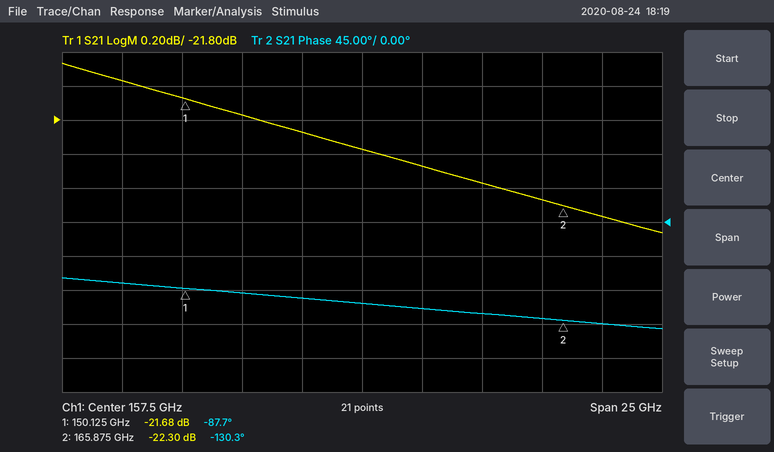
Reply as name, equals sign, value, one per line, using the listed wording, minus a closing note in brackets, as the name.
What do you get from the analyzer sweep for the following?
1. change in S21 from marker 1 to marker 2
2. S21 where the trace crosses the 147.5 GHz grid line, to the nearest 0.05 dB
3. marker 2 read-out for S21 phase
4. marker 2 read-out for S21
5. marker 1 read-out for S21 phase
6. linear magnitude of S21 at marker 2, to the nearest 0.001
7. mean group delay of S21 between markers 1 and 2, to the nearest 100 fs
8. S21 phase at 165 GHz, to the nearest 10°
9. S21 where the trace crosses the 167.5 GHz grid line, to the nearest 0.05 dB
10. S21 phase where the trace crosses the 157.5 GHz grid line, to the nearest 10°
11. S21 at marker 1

change in S21 from marker 1 to marker 2 = -0.62 dB
S21 where the trace crosses the 147.5 GHz grid line, to the nearest 0.05 dB = -21.55 dB
marker 2 read-out for S21 phase = -130.3°
marker 2 read-out for S21 = -22.30 dB
marker 1 read-out for S21 phase = -87.7°
linear magnitude of S21 at marker 2, to the nearest 0.001 = 0.077
mean group delay of S21 between markers 1 and 2, to the nearest 100 fs = 7.5 ps
S21 phase at 165 GHz, to the nearest 10° = -130°
S21 where the trace crosses the 167.5 GHz grid line, to the nearest 0.05 dB = -22.35 dB
S21 phase where the trace crosses the 157.5 GHz grid line, to the nearest 10° = -110°
S21 at marker 1 = -21.68 dB
